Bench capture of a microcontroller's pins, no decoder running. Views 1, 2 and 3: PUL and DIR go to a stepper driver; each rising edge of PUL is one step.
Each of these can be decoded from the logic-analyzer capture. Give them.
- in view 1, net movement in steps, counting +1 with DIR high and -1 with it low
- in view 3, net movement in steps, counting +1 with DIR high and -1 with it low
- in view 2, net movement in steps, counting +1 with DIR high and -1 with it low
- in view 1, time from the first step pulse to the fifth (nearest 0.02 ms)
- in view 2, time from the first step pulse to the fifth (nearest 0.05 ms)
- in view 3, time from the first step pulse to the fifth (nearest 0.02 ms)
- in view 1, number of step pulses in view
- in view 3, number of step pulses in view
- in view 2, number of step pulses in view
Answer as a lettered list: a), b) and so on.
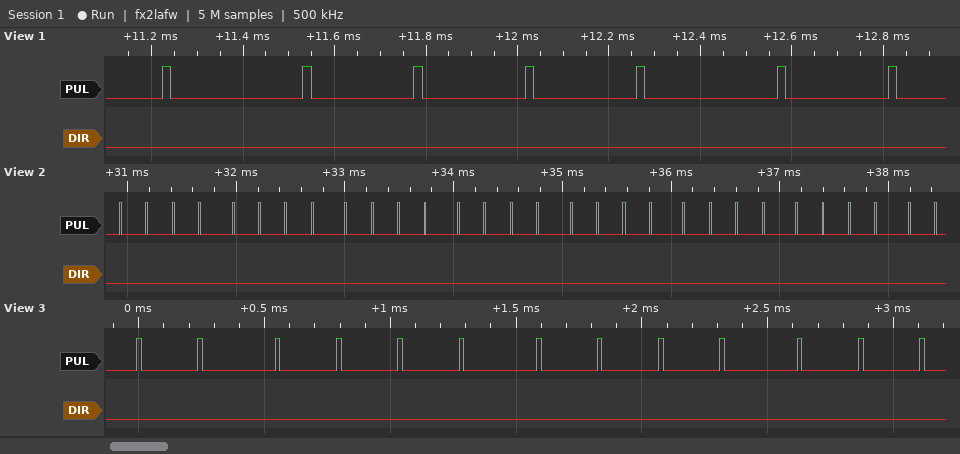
a) -7
b) -13
c) -30
d) 1.04 ms
e) 1.05 ms
f) 1.04 ms
g) 7
h) 13
i) 30
